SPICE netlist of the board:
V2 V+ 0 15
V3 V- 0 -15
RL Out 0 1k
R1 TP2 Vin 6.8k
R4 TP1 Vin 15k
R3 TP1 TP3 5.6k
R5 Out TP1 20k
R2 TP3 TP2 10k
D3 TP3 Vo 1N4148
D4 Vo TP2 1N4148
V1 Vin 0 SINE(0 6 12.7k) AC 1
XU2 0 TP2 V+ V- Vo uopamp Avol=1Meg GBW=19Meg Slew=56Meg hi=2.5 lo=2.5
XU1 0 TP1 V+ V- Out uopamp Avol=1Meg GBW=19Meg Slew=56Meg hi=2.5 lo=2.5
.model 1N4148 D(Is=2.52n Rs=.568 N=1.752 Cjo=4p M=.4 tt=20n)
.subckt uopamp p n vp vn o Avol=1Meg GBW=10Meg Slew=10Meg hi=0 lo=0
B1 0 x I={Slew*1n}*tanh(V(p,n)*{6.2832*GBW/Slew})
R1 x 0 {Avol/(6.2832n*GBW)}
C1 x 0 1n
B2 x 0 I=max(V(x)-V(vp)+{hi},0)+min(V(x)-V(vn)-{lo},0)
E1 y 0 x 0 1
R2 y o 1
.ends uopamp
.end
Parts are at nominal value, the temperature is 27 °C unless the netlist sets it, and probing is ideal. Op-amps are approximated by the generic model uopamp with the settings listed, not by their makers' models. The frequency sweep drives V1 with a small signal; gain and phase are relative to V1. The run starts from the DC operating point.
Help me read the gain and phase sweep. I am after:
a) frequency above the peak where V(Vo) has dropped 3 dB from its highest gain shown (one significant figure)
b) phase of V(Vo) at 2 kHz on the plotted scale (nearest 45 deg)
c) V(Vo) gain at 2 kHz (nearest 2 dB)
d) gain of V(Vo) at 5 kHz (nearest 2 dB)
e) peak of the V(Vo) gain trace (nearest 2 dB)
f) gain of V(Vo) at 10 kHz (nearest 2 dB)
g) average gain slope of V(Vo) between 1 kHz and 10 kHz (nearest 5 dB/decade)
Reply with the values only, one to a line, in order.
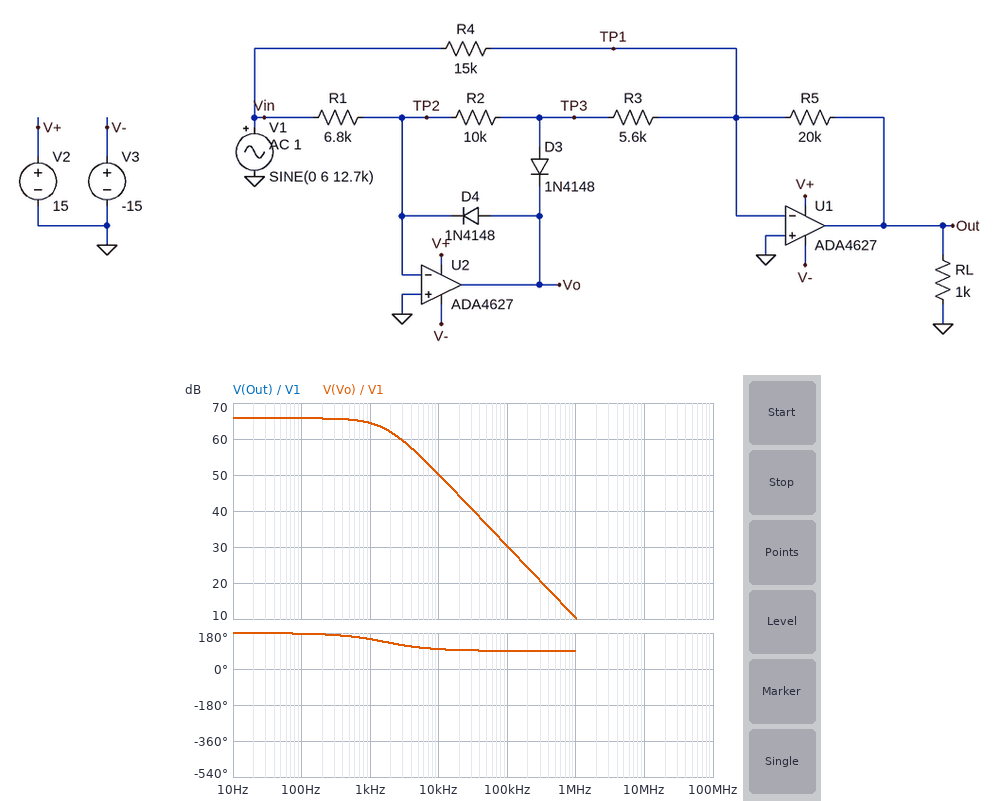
2 kHz
135 deg
62 dB
56 dB
66 dB
50 dB
-15 dB/decade
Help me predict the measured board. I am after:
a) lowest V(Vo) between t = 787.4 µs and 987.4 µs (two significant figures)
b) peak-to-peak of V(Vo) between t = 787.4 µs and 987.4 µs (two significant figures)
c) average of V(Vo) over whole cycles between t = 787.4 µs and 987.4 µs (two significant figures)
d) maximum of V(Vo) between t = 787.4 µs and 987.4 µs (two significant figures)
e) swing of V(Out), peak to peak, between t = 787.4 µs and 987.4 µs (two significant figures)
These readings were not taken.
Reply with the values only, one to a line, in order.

-9.4 V
10 V
-2.8 V
580 mV
13 V
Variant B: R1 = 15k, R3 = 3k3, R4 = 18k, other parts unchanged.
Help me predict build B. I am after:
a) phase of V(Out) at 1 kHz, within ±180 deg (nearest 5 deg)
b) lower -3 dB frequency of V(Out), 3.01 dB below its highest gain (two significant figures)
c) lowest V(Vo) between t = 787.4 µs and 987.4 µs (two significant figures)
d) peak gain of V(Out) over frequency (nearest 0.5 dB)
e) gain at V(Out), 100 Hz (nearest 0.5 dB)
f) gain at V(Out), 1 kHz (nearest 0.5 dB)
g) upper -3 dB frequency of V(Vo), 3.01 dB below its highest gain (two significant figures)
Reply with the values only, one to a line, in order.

-160 deg
1.2 kHz
-4.6 V
-4.5 dB
-10.0 dB
-8.0 dB
1.8 kHz
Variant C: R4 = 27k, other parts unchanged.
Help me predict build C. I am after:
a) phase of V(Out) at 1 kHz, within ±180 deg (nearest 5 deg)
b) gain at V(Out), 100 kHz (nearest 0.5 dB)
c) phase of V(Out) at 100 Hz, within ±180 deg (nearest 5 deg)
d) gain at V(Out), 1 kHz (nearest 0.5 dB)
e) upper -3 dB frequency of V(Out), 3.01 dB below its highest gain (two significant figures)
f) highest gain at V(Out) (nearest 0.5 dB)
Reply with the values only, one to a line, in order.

-25 deg
-21.0 dB
-5 deg
-5.0 dB
1.7 kHz
-4.0 dB
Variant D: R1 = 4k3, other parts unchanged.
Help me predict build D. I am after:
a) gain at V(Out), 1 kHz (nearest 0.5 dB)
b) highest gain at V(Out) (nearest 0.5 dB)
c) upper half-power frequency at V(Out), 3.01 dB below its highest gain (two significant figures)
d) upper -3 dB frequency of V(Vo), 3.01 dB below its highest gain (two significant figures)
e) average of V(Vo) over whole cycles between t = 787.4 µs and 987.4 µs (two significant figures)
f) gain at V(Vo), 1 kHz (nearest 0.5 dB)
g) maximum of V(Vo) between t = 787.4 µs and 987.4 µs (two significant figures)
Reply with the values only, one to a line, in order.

-3.0 dB
-1.5 dB
1.6 kHz
1.5 kHz
-4.2 V
68.0 dB
600 mV
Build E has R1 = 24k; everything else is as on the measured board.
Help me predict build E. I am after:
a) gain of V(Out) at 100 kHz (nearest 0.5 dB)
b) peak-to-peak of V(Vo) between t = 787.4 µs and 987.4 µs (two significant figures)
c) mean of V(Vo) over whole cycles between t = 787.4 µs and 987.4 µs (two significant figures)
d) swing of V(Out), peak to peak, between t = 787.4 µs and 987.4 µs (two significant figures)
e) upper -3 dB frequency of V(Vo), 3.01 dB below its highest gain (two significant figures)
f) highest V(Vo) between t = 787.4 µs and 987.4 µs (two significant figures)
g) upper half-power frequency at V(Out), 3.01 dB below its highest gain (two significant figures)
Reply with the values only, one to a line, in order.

0.5 dB
3.6 V
-820 mV
8.3 V
1.9 kHz
520 mV
5.7 MHz
